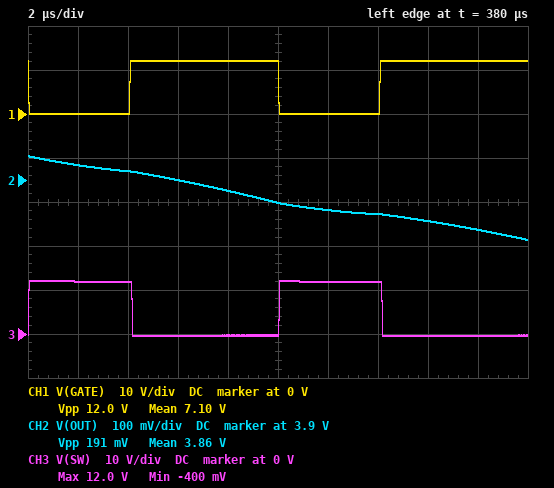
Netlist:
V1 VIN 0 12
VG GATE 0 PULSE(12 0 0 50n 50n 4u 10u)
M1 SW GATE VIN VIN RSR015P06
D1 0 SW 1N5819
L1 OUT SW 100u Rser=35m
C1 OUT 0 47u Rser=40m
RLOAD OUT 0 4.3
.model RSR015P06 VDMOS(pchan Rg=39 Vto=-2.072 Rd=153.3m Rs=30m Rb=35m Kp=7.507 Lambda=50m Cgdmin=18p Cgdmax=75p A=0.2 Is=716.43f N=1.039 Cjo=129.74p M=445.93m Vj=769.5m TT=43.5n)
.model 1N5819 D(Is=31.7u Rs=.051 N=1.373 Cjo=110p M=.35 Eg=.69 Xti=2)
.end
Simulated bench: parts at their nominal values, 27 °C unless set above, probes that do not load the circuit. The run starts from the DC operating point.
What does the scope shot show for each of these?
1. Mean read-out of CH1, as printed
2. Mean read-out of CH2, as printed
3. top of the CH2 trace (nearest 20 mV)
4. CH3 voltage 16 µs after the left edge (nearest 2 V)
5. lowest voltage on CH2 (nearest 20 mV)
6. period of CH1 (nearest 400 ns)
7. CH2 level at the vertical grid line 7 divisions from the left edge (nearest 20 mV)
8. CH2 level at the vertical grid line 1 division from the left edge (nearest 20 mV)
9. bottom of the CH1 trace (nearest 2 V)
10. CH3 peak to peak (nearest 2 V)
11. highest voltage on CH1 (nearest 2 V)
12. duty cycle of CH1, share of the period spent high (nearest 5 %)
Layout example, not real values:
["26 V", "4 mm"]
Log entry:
["7.10 V", "3.86 V", "3.96 V", "0 V", "3.76 V", "10.0 µs", "3.82 V", "3.94 V", "0 V", "12 V", "12 V", "60 %"]
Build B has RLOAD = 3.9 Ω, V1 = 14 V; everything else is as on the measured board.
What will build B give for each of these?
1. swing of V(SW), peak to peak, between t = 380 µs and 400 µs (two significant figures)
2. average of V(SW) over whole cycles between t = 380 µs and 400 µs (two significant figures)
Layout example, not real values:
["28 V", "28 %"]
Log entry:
["14 V", "5.7 V"]
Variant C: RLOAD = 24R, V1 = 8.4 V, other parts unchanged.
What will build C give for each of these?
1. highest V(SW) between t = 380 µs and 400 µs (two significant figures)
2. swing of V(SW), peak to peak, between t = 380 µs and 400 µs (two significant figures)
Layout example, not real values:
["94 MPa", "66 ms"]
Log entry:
["9.0 V", "9.3 V"]
